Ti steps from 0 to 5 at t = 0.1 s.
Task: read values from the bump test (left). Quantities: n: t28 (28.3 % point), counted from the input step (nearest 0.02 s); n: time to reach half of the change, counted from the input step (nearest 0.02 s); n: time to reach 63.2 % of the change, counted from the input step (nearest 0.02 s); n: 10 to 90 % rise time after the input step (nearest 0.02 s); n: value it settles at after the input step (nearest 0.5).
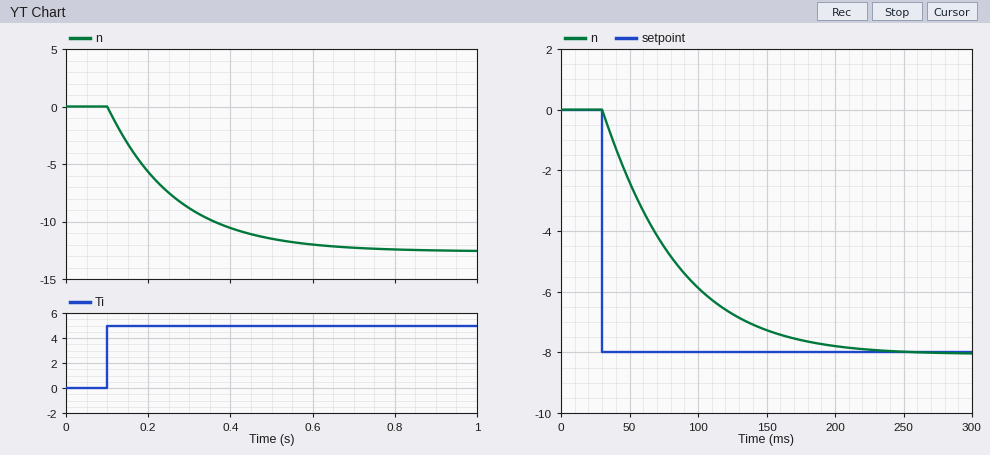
0.06 s
0.12 s
0.16 s
0.36 s
-12.5
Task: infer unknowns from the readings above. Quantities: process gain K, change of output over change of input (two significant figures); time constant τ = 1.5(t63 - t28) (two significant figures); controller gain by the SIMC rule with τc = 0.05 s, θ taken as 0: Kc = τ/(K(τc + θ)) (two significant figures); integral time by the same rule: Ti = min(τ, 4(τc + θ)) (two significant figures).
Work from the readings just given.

-2.5
0.15 s
-1.2
0.15 s
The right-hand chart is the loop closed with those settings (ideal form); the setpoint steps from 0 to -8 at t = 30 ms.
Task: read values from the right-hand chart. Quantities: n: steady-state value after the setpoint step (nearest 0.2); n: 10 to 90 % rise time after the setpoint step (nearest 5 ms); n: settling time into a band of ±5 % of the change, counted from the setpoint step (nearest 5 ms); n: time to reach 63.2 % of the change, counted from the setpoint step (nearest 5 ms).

-8.0
110 ms
145 ms
55 ms
